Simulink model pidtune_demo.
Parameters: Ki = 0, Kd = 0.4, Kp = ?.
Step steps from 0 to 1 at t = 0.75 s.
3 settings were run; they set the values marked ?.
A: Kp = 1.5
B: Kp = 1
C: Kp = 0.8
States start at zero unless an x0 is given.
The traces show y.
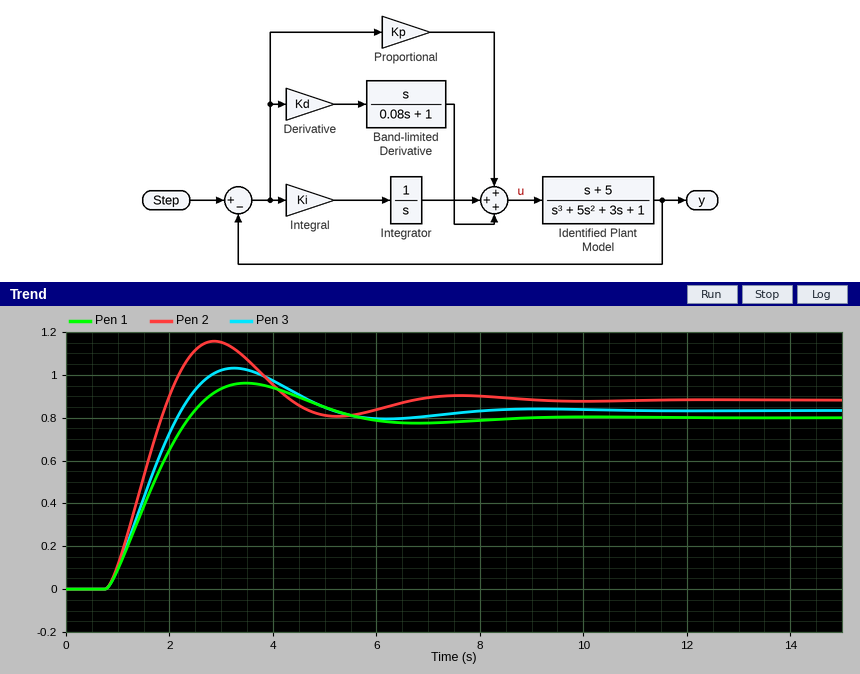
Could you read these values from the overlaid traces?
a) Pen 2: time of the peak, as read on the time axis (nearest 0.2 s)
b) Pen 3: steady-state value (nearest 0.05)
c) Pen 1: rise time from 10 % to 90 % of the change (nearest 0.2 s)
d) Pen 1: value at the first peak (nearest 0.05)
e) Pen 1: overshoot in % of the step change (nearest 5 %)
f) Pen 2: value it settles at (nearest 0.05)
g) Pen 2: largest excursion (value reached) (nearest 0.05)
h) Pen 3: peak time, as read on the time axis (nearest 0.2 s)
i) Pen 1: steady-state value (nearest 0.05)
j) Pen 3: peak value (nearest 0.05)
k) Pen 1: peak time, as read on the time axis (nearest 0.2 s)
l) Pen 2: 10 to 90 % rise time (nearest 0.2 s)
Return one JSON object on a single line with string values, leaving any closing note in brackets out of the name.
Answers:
{"Pen 2: time of the peak, as read on the time axis": "2.8 s", "Pen 3: steady-state value": "0.85", "Pen 1: rise time from 10 % to 90 % of the change": "1.2 s", "Pen 1: value at the first peak": "0.95", "Pen 1: overshoot in % of the step change": "20 %", "Pen 2: value it settles at": "0.90", "Pen 2: largest excursion (value reached)": "1.15", "Pen 3: peak time, as read on the time axis": "3.2 s", "Pen 1: steady-state value": "0.80", "Pen 3: peak value": "1.05", "Pen 1: peak time, as read on the time axis": "3.4 s", "Pen 2: 10 to 90 % rise time": "0.8 s"}
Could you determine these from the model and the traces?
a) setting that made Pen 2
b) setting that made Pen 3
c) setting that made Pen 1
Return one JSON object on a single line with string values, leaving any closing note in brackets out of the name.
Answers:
{"setting that made Pen 2": "A", "setting that made Pen 3": "B", "setting that made Pen 1": "C"}
